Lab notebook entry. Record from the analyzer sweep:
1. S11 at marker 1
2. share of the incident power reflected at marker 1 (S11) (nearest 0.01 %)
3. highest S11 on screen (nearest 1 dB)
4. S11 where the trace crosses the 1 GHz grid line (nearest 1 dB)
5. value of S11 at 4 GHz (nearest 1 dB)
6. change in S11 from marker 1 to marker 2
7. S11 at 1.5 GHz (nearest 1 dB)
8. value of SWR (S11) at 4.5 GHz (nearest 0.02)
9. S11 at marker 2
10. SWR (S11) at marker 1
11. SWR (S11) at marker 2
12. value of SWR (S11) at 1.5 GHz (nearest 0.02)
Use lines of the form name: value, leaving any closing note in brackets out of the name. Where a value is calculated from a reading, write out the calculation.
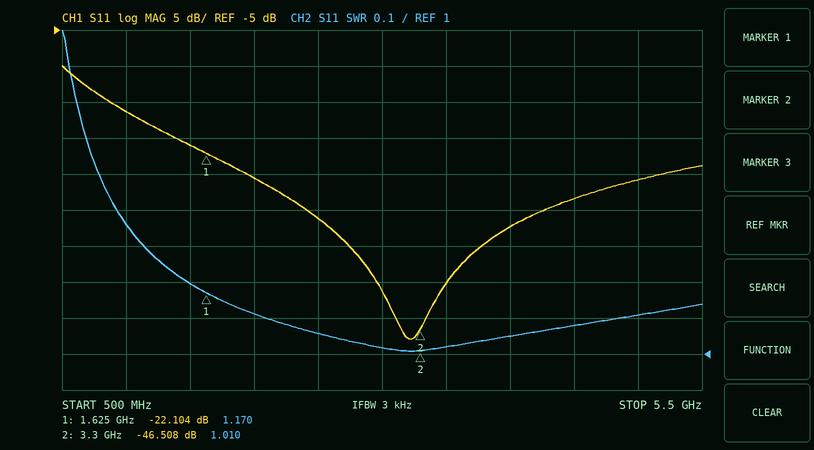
S11 at marker 1: -22.104 dB
share of the incident power reflected at marker 1 (S11): 10^(-22.104/10) ≈ 0.62 %
highest S11 on screen: -10 dB
S11 where the trace crosses the 1 GHz grid line: -16 dB
value of S11 at 4 GHz: -32 dB
change in S11 from marker 1 to marker 2: -46.508 − (-22.104) = -24.404 dB
S11 at 1.5 GHz: -21 dB
value of SWR (S11) at 4.5 GHz: 1.08
S11 at marker 2: -46.508 dB
SWR (S11) at marker 1: 1.170
SWR (S11) at marker 2: 1.010
value of SWR (S11) at 1.5 GHz: 1.20
